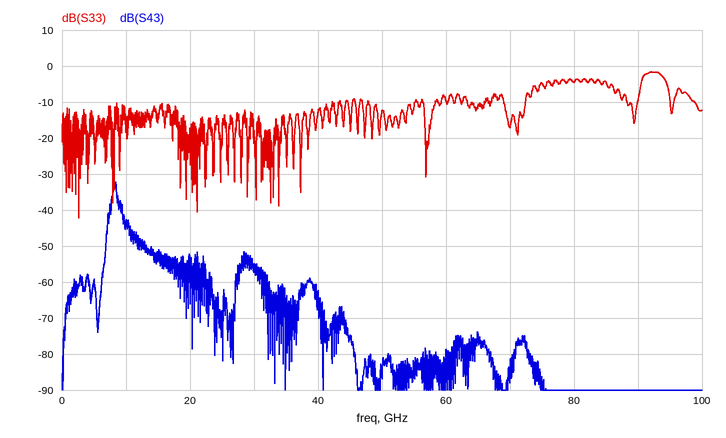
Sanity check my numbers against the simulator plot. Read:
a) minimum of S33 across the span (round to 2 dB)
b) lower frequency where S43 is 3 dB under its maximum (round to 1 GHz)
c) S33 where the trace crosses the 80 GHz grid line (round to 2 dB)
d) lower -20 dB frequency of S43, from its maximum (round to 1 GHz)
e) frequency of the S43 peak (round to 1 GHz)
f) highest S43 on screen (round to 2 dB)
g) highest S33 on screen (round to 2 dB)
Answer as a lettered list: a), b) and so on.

a) -42 dB
b) 8 GHz
c) -4 dB
d) 7 GHz
e) 8 GHz
f) -32 dB
g) -2 dB
